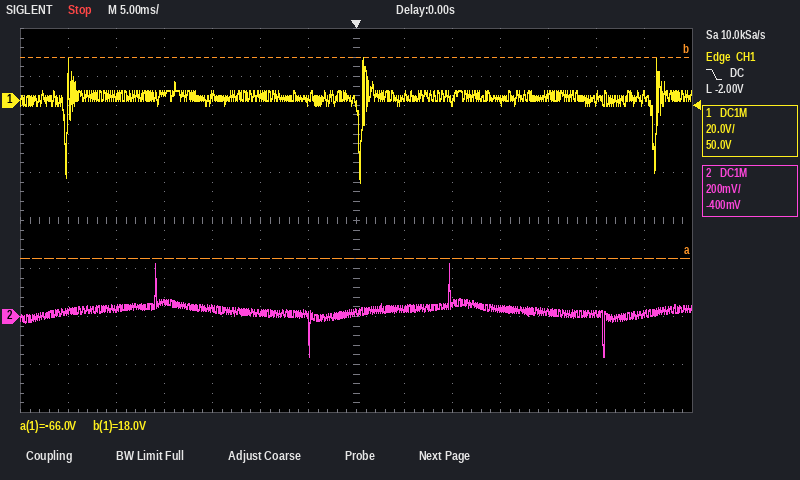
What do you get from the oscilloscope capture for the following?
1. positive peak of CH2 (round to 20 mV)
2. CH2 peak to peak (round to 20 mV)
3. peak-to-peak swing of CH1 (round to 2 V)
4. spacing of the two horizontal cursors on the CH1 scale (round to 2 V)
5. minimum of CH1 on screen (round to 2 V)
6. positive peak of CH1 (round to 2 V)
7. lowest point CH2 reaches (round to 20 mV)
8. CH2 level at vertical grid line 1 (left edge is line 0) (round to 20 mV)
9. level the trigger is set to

220 mV
380 mV
52 V
84 V
-34 V
18 V
-160 mV
20 mV
-2.00 V
